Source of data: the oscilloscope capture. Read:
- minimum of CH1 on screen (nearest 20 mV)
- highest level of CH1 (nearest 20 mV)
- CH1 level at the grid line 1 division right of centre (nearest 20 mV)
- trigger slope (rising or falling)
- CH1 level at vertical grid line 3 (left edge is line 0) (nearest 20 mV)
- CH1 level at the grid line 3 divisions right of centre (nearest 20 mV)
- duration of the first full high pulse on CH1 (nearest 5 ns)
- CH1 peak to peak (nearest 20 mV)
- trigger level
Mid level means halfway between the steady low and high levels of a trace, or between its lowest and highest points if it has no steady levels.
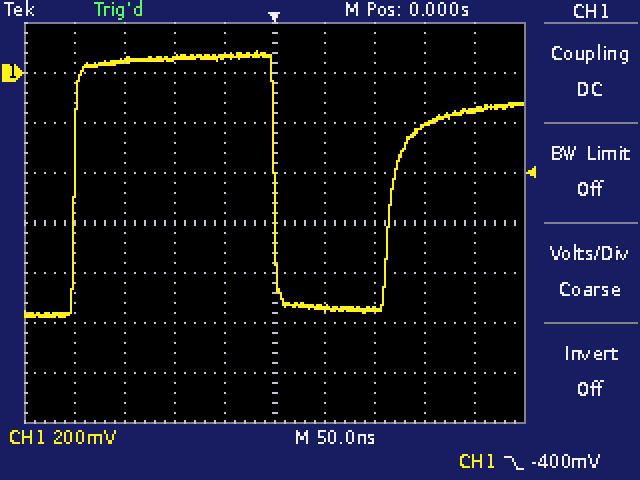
-980 mV
80 mV
-940 mV
falling
60 mV
-220 mV
200 ns
1.06 V
-400 mV
